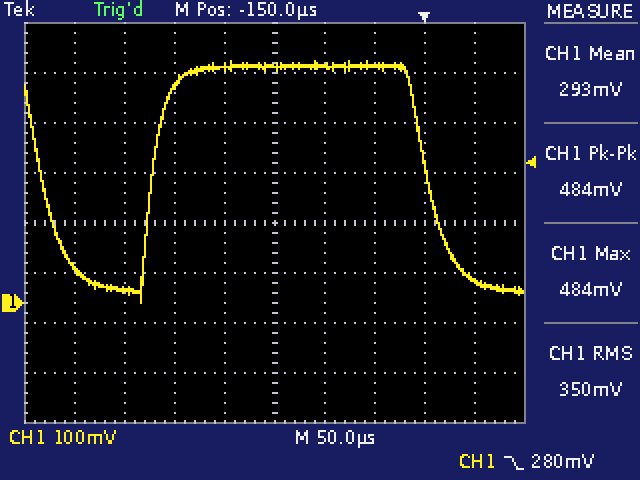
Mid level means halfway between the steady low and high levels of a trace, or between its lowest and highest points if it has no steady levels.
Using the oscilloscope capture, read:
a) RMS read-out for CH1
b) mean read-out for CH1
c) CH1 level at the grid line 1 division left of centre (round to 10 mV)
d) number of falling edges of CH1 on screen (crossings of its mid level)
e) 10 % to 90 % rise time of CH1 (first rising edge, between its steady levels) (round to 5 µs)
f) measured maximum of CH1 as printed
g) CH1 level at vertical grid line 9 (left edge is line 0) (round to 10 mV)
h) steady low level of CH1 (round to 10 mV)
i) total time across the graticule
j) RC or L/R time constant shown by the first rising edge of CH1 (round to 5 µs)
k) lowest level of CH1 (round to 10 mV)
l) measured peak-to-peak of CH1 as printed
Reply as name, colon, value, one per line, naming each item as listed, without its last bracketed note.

RMS read-out for CH1: 350 mV
mean read-out for CH1: 293 mV
CH1 level at the grid line 1 division left of centre: 470 mV
number of falling edges of CH1 on screen: 2
10 % to 90 % rise time of CH1 (first rising edge, between its steady levels): 30 µs
measured maximum of CH1 as printed: 484 mV
CH1 level at vertical grid line 9 (left edge is line 0): 40 mV
steady low level of CH1: 30 mV
total time across the graticule: 500 µs
RC or L/R time constant shown by the first rising edge of CH1: 15 µs
lowest level of CH1: 0 mV
measured peak-to-peak of CH1 as printed: 484 mV
